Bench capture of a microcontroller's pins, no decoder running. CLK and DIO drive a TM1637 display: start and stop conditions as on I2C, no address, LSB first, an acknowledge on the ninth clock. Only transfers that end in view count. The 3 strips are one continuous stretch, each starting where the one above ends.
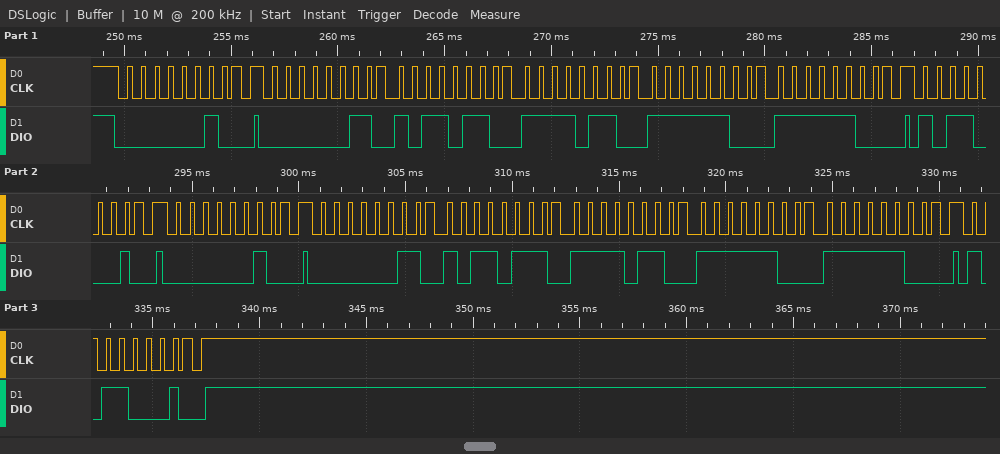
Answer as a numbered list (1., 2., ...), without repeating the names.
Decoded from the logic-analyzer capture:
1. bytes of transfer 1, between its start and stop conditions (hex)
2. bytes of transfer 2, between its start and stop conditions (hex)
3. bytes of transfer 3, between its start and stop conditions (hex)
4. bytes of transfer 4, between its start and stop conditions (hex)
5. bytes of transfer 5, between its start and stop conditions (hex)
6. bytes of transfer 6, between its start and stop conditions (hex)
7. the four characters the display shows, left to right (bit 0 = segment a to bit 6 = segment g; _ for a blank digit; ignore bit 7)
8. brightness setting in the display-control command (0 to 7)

1. 40
2. C0 6D 6F 3F 3F
3. 8D
4. 40
5. C0 ED 6F 3F 3F
6. 8D
7. 5900
8. 5
